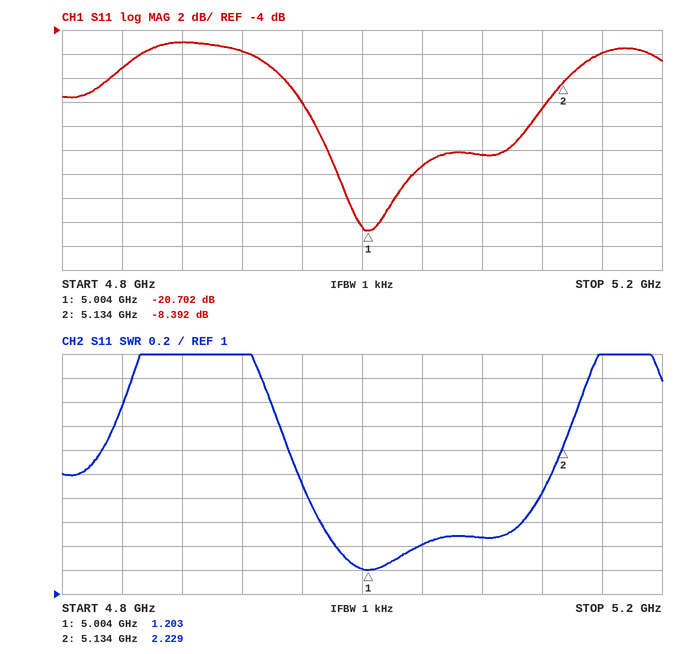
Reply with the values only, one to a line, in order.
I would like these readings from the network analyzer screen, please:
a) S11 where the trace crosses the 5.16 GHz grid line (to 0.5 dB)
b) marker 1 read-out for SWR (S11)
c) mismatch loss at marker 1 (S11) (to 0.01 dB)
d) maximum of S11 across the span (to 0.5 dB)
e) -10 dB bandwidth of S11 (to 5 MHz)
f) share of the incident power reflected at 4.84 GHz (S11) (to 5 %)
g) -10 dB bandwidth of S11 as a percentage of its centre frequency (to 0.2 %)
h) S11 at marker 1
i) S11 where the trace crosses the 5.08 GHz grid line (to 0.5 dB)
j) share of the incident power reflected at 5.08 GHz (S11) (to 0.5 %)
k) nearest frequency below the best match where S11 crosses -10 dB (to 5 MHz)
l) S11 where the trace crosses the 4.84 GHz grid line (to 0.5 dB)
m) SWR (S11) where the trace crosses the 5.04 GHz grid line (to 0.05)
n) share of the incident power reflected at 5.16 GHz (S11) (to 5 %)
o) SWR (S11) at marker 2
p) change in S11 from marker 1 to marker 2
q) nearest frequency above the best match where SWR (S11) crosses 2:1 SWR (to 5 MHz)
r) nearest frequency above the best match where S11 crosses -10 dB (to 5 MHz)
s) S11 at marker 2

-6.0 dB
1.203
0.04 dB
-5.0 dB
165 MHz
20 %
3.2 %
-20.702 dB
-14.5 dB
3.5 %
4.960 GHz
-7.0 dB
1.40
25 %
2.229
12.310 dB
5.125 GHz
5.125 GHz
-8.392 dB
